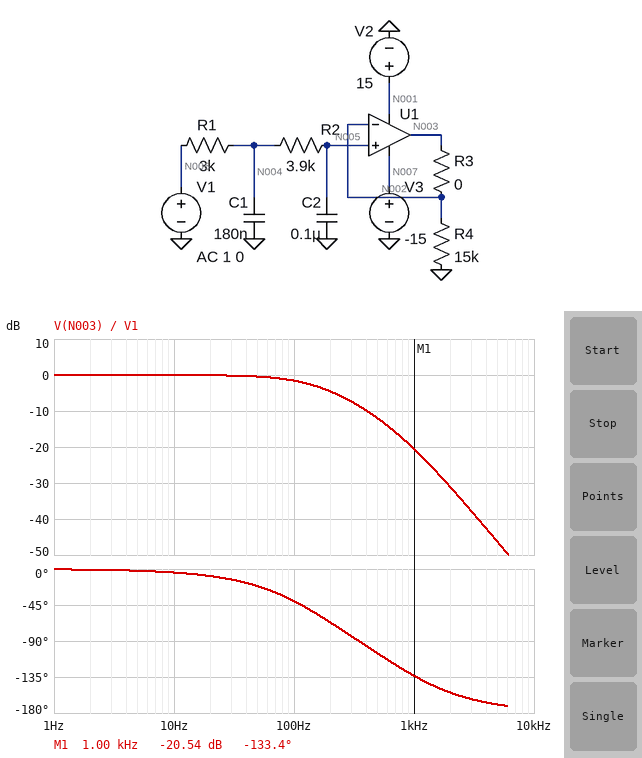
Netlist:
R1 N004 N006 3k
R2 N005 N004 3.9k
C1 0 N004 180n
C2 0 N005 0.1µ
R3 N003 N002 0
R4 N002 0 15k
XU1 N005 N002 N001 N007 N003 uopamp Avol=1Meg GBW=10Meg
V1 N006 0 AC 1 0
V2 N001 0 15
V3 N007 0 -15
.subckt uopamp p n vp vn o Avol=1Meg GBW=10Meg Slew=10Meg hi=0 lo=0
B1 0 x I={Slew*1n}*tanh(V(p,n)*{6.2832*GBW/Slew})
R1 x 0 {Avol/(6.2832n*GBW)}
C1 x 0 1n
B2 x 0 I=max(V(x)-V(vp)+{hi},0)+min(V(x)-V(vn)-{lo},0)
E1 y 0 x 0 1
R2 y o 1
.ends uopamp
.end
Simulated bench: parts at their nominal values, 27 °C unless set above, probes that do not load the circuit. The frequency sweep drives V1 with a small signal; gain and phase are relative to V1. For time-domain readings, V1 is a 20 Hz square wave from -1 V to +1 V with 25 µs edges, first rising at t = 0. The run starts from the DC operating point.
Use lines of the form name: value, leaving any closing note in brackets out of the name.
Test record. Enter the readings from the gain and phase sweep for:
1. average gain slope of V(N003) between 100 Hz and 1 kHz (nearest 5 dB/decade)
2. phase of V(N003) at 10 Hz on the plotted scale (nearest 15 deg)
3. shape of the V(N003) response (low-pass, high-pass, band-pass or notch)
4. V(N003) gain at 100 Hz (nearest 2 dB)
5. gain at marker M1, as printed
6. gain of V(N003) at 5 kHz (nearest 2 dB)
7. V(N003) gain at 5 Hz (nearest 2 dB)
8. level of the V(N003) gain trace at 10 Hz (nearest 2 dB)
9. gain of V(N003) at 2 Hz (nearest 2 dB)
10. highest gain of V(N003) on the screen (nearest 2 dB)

average gain slope of V(N003) between 100 Hz and 1 kHz: -20 dB/decade
phase of V(N003) at 10 Hz on the plotted scale: 0 deg
shape of the V(N003) response: low-pass
V(N003) gain at 100 Hz: -2 dB
gain at marker M1, as printed: -20.54 dB
gain of V(N003) at 5 kHz: -46 dB
V(N003) gain at 5 Hz: 0 dB
level of the V(N003) gain trace at 10 Hz: 0 dB
gain of V(N003) at 2 Hz: 0 dB
highest gain of V(N003) on the screen: 0 dB
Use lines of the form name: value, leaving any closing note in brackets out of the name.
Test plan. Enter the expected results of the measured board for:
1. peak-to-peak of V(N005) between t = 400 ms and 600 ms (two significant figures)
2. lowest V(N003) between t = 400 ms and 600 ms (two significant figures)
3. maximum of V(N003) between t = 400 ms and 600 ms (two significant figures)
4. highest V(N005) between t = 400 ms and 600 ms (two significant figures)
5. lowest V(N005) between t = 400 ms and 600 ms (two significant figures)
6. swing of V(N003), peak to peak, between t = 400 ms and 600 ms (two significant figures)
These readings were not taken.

peak-to-peak of V(N005) between t = 400 ms and 600 ms: 2.0 V
lowest V(N003) between t = 400 ms and 600 ms: -1.0 V
maximum of V(N003) between t = 400 ms and 600 ms: 1.0 V
highest V(N005) between t = 400 ms and 600 ms: 1.0 V
lowest V(N005) between t = 400 ms and 600 ms: -1.0 V
swing of V(N003), peak to peak, between t = 400 ms and 600 ms: 2.0 V
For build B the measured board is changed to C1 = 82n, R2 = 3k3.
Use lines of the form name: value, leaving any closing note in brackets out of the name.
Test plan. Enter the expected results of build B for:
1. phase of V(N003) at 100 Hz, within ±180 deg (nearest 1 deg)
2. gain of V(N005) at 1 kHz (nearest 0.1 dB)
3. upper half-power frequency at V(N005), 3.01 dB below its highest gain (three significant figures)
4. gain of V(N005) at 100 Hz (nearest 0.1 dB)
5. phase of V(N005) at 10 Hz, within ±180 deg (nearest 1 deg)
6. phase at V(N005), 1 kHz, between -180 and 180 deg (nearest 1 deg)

phase of V(N003) at 100 Hz, within ±180 deg: -30 deg
gain of V(N005) at 1 kHz: -15.5 dB
upper half-power frequency at V(N005), 3.01 dB below its highest gain: 203 Hz
gain of V(N005) at 100 Hz: -0.9 dB
phase of V(N005) at 10 Hz, within ±180 deg: -3 deg
phase at V(N005), 1 kHz, between -180 and 180 deg: -112 deg
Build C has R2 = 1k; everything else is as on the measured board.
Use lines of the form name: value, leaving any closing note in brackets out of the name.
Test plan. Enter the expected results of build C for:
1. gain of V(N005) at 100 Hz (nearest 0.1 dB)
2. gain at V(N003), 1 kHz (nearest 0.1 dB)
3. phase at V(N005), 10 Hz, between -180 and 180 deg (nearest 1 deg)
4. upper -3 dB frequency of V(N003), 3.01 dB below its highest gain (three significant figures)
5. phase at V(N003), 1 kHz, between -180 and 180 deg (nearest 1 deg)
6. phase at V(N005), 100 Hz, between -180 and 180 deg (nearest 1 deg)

gain of V(N005) at 100 Hz: -1.2 dB
gain at V(N003), 1 kHz: -15.6 dB
phase at V(N005), 10 Hz, between -180 and 180 deg: -3 deg
upper -3 dB frequency of V(N003), 3.01 dB below its highest gain: 180 Hz
phase at V(N003), 1 kHz, between -180 and 180 deg: -101 deg
phase at V(N005), 100 Hz, between -180 and 180 deg: -31 deg
